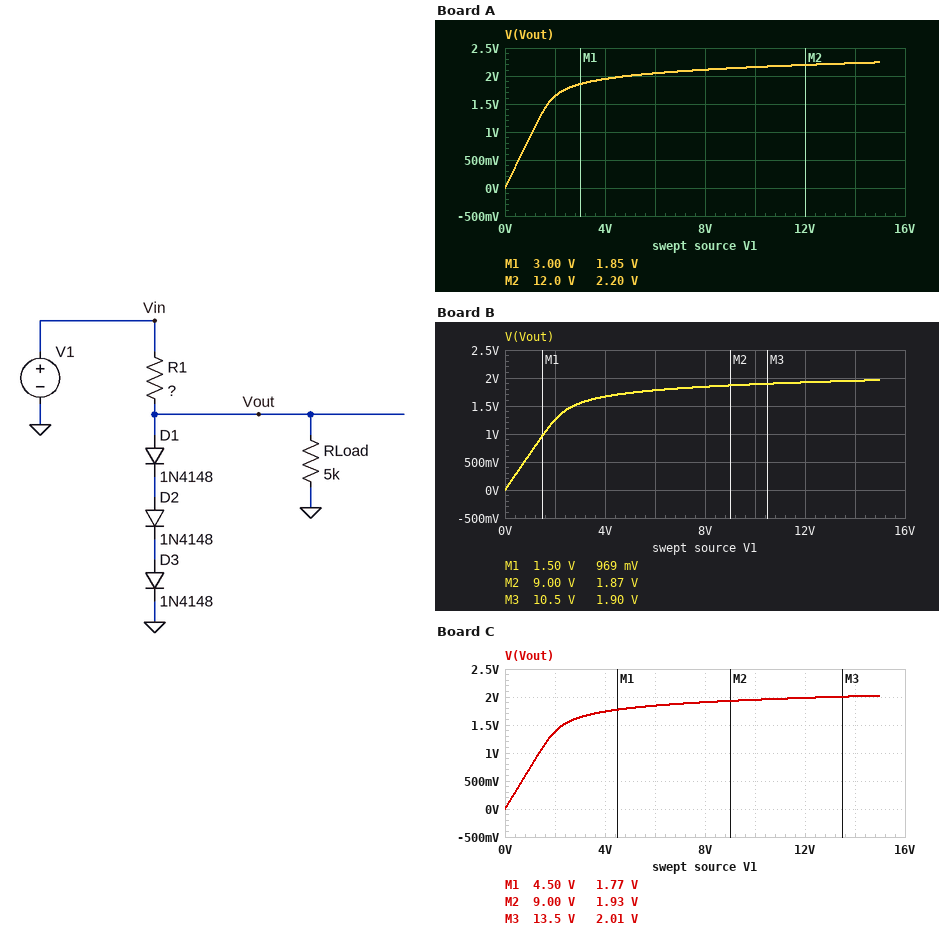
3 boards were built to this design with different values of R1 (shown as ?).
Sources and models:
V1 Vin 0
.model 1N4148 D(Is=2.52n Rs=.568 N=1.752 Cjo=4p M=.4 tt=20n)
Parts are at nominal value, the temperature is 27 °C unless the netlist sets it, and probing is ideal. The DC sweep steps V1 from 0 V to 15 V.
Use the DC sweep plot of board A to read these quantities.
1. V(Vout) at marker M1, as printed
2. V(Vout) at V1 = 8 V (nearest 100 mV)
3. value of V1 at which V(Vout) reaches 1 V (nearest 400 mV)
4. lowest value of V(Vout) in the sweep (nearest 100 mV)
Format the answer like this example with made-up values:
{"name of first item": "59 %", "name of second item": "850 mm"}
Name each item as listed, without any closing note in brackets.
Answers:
{"V(Vout) at marker M1, as printed": "1.85 V", "V(Vout) at V1 = 8 V": "2.1 V", "value of V1 at which V(Vout) reaches 1 V": "1.2 V", "lowest value of V(Vout) in the sweep": "0 V"}
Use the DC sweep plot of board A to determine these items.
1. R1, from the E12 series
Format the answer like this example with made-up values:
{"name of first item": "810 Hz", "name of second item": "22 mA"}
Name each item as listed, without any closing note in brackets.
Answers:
{"R1, from the E12 series": "470 Ω"}
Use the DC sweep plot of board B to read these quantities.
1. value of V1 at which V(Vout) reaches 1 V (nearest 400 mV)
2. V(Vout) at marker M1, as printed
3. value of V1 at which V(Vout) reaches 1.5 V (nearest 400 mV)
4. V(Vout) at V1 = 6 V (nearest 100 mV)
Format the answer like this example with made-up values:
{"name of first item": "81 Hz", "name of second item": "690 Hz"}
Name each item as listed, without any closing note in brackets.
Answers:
{"value of V1 at which V(Vout) reaches 1 V": "1.6 V", "V(Vout) at marker M1, as printed": "969 mV", "value of V1 at which V(Vout) reaches 1.5 V": "2.8 V", "V(Vout) at V1 = 6 V": "1.8 V"}
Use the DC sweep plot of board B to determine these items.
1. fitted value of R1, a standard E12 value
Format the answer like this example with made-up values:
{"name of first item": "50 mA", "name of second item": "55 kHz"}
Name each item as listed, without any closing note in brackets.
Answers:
{"fitted value of R1, a standard E12 value": "2.7 kΩ"}
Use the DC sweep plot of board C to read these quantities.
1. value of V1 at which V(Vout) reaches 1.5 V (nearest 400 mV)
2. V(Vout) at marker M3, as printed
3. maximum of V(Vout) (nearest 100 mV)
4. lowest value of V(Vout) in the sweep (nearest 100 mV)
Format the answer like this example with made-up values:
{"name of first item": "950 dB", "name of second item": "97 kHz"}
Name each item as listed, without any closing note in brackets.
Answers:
{"value of V1 at which V(Vout) reaches 1.5 V": "2.4 V", "V(Vout) at marker M3, as printed": "2.01 V", "maximum of V(Vout)": "2.0 V", "lowest value of V(Vout) in the sweep": "0 V"}
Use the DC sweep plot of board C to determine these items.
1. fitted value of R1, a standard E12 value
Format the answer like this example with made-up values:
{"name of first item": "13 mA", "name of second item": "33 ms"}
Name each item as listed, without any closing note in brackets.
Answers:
{"fitted value of R1, a standard E12 value": "1.8 kΩ"}
